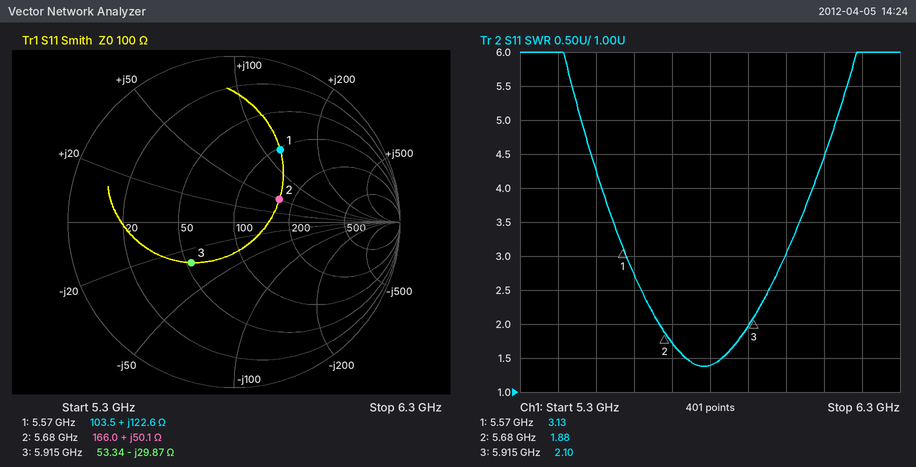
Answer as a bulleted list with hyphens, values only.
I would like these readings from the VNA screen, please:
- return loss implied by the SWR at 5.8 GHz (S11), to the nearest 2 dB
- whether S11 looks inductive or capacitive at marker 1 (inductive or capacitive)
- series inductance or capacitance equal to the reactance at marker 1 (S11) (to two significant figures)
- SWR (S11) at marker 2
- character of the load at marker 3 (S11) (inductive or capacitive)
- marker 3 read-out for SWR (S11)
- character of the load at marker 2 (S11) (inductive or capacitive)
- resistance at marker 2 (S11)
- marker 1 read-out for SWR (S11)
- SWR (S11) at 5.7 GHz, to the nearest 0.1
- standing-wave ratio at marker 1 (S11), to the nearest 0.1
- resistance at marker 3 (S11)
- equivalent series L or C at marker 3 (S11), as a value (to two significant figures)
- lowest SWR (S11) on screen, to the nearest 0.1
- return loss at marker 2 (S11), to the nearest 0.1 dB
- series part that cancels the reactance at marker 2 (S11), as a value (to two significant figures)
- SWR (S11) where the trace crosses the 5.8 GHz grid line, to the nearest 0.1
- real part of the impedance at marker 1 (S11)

- 16 dB
- inductive
- 3.5 nH
- 1.88
- capacitive
- 2.10
- inductive
- 166.0 Ω
- 3.13
- 1.7
- 3.1
- 53.34 Ω
- 900 fF
- 1.4
- 10.3 dB
- 560 fF
- 1.4
- 103.5 Ω
